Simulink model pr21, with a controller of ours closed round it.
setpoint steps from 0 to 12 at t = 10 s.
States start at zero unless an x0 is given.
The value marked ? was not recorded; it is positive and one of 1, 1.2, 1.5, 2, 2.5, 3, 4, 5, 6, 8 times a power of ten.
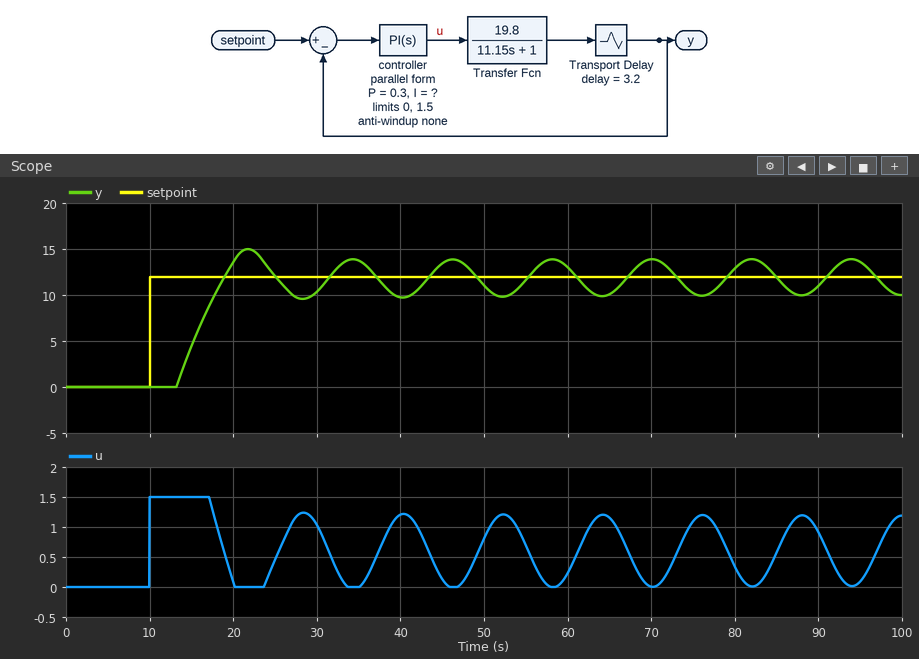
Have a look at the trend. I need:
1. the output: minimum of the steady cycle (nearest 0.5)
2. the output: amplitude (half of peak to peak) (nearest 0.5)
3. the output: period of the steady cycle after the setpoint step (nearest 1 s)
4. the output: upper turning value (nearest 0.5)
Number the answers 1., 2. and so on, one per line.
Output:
1. 10.0
2. 2.0
3. 12 s
4. 14.0
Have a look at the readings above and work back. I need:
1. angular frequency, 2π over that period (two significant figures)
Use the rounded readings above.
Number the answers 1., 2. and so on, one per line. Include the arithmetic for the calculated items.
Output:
1. 2π / 12 = 0.52 rad/s
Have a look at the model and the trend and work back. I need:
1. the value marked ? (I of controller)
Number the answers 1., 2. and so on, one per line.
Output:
1. 0.008
